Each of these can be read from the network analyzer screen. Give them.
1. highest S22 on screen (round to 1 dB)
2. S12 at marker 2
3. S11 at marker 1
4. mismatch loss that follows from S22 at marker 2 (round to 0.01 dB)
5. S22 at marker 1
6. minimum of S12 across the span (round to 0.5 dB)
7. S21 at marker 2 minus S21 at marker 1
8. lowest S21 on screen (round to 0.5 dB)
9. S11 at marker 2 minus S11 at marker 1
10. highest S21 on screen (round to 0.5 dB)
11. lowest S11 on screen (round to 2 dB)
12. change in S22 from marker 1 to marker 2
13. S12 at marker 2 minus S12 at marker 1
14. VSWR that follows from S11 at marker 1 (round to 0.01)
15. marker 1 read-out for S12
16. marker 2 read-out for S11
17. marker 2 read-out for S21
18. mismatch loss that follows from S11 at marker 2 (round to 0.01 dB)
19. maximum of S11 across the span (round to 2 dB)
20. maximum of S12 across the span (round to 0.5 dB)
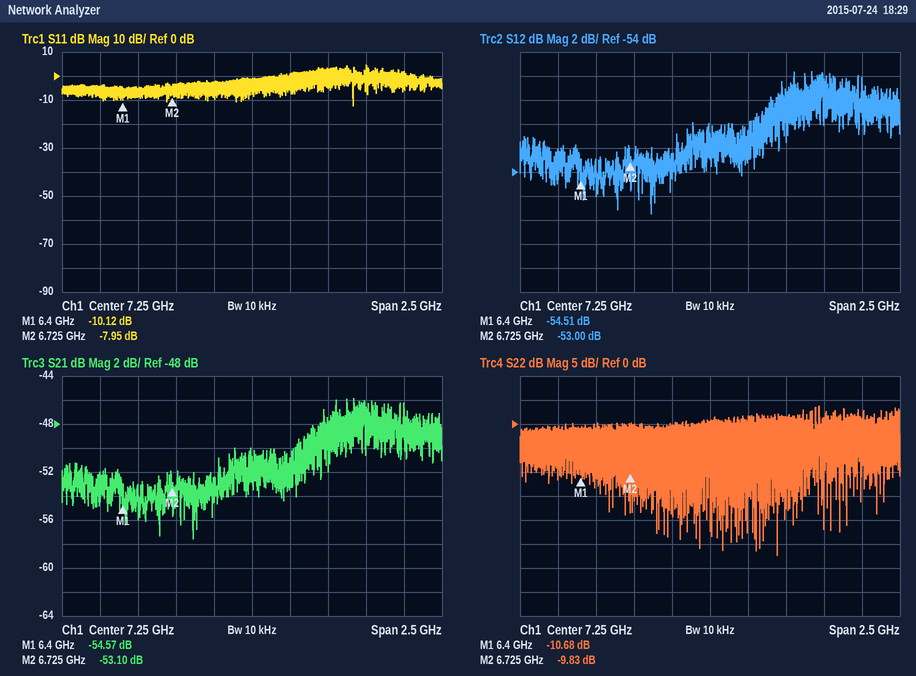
4 dB
-53.00 dB
-10.12 dB
0.48 dB
-10.68 dB
-57.5 dB
1.47 dB
-57.5 dB
2.17 dB
-46.0 dB
-12 dB
0.85 dB
1.51 dB
1.91
-54.51 dB
-7.95 dB
-53.10 dB
0.76 dB
4 dB
-45.5 dB
